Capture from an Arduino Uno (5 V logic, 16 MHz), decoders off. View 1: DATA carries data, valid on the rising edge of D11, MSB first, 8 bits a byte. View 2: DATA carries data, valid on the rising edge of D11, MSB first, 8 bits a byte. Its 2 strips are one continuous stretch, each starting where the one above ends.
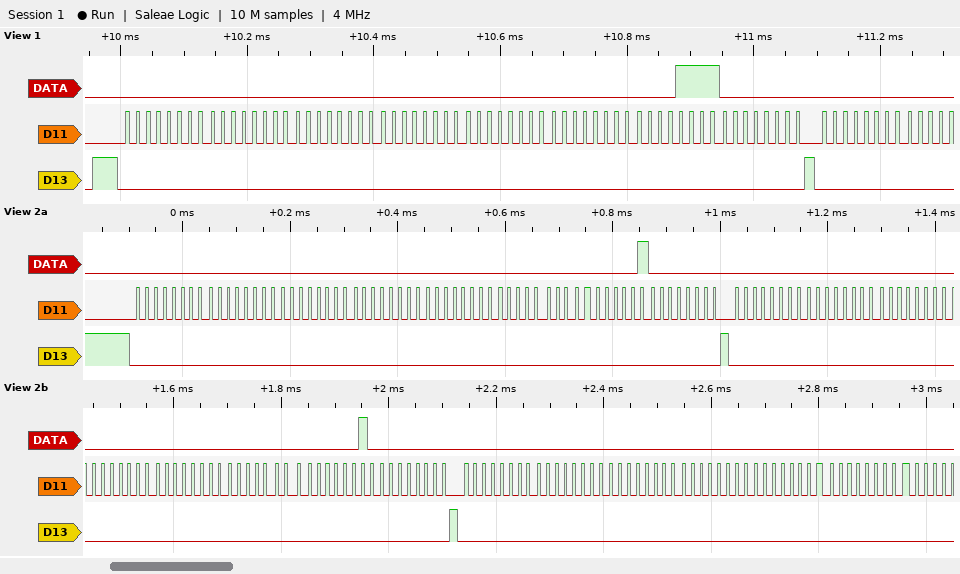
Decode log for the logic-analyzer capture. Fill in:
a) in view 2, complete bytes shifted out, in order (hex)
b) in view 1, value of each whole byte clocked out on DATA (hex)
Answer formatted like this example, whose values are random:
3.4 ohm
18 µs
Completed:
0x00 0x00 0x00 0x00 0x00 0x00 0x01 0x00 0x00 0x00 0x00 0x00 0x00 0x00 0x02 0x00 0x00 0x00 0x00 0x00 0x00 0x00
00 00 00 00 00 00 0F 00 00
